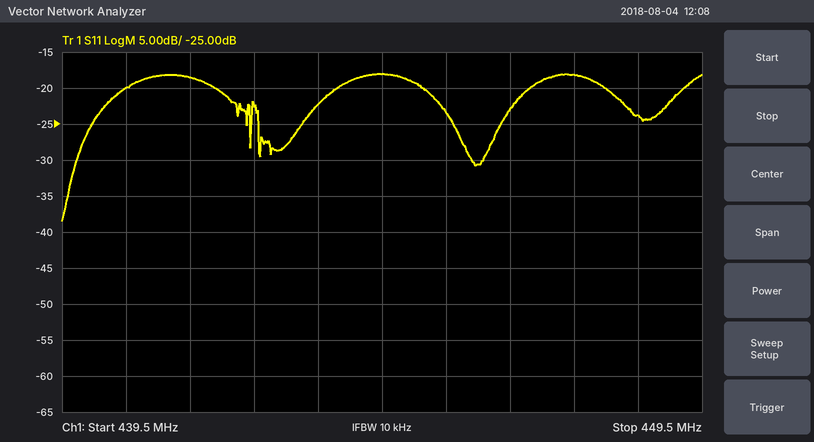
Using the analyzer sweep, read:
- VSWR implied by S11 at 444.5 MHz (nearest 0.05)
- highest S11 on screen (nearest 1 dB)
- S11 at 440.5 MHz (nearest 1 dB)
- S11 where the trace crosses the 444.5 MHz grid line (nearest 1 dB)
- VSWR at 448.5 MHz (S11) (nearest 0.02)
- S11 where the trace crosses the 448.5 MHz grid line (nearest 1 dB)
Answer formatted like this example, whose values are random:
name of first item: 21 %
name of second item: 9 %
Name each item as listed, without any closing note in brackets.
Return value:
VSWR implied by S11 at 444.5 MHz: 1.30
highest S11 on screen: -18 dB
S11 at 440.5 MHz: -20 dB
S11 where the trace crosses the 444.5 MHz grid line: -18 dB
VSWR at 448.5 MHz (S11): 1.14
S11 where the trace crosses the 448.5 MHz grid line: -24 dB
